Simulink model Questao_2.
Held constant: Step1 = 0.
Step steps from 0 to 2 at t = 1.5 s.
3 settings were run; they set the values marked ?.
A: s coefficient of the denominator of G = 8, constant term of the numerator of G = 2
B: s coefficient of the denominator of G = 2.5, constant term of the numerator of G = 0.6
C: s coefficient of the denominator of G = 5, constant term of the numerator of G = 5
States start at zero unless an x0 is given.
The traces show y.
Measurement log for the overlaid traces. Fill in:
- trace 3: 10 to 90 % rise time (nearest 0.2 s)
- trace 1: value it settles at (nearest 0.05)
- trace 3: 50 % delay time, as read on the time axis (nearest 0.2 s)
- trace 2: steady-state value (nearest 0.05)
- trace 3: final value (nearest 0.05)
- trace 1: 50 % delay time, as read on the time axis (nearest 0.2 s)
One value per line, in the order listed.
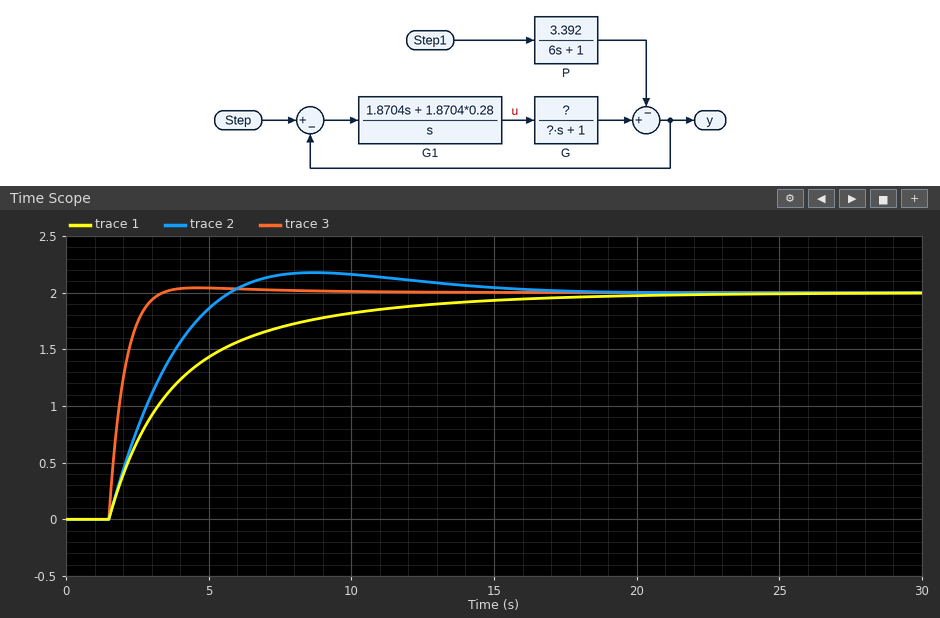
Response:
1.0 s
2.00
1.8 s
2.00
2.00
3.2 s
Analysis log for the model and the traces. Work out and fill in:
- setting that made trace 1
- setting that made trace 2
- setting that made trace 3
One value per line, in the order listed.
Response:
B
A
C
